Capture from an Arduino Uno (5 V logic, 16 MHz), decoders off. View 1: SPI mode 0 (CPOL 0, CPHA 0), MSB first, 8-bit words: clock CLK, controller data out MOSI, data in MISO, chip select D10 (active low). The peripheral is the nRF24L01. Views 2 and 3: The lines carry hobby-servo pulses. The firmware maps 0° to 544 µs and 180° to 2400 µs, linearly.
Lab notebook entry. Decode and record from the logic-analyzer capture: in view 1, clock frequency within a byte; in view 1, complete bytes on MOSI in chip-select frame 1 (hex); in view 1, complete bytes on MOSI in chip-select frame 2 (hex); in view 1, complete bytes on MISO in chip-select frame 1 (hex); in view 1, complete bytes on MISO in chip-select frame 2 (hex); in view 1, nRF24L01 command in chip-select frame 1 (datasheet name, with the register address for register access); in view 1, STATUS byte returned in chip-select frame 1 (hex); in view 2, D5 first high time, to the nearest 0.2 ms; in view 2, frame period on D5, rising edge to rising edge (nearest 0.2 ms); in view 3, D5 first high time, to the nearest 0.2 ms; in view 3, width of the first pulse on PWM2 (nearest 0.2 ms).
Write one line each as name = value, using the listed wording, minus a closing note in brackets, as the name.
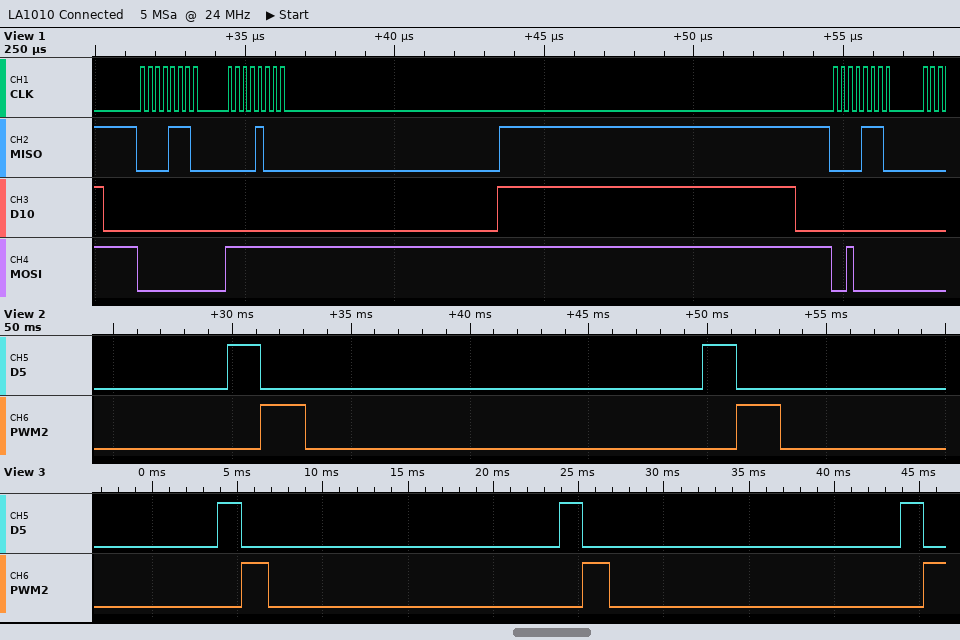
in view 1, clock frequency within a byte = 4 MHz
in view 1, complete bytes on MOSI in chip-select frame 1 = 00 FF
in view 1, complete bytes on MOSI in chip-select frame 2 = 20
in view 1, complete bytes on MISO in chip-select frame 1 = 0E 08
in view 1, complete bytes on MISO in chip-select frame 2 = 0E
in view 1, nRF24L01 command in chip-select frame 1 = R_REGISTER 0x00
in view 1, STATUS byte returned in chip-select frame 1 = 0x0E
in view 2, D5 first high time, to the nearest 0.2 ms = 1.4 ms
in view 2, frame period on D5, rising edge to rising edge = 20.0 ms
in view 3, D5 first high time, to the nearest 0.2 ms = 1.4 ms
in view 3, width of the first pulse on PWM2 = 1.6 ms
